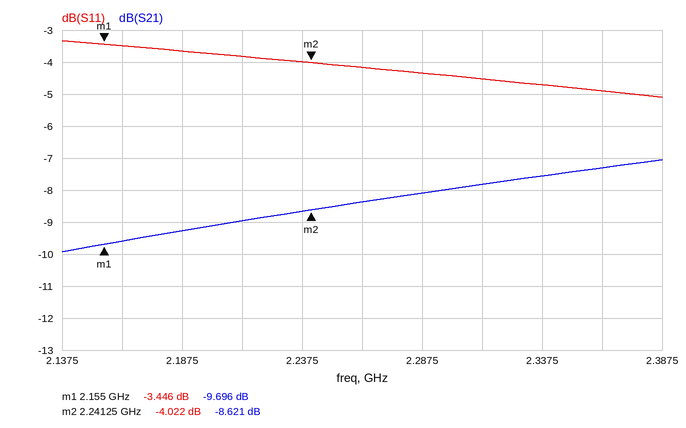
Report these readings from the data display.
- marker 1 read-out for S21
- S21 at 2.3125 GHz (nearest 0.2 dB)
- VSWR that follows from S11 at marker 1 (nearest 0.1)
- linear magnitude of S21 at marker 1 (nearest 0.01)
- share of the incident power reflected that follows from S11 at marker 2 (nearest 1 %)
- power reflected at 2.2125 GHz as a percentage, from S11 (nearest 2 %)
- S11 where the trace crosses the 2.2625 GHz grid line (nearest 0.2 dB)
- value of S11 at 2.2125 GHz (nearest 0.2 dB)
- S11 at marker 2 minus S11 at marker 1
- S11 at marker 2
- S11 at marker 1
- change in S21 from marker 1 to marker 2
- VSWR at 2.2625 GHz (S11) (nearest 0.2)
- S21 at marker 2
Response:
-9.696 dB
-7.8 dB
5.1
0.33
40 %
42 %
-4.2 dB
-3.8 dB
-0.576 dB
-4.022 dB
-3.446 dB
1.075 dB
4.2
-8.621 dB
